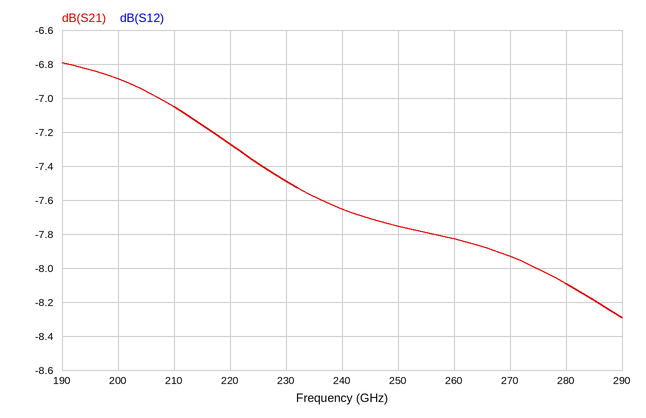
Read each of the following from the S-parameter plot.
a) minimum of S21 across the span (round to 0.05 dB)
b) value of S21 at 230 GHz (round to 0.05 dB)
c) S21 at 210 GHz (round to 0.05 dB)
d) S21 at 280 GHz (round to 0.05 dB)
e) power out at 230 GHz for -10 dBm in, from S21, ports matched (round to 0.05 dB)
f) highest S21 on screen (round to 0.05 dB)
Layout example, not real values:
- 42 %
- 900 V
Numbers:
- -8.30 dB
- -7.50 dB
- -7.05 dB
- -8.10 dB
- -17.50 dBm
- -6.80 dB
